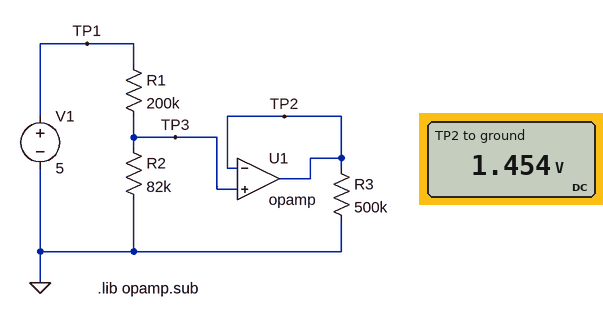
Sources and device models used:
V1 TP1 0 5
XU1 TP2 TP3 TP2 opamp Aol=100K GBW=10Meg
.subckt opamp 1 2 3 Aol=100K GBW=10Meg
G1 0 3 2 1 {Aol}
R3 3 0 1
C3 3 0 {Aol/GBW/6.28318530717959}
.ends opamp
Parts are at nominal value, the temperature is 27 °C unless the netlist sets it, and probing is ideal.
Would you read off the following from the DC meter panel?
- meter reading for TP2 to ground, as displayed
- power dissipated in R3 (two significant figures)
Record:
1.454 V
4.2 µW
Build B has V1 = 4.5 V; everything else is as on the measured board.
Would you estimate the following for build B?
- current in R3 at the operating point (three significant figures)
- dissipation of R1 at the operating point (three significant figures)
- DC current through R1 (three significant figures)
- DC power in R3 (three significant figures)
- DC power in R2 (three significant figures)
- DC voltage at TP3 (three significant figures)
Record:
2.62 µA
50.9 µW
16.0 µA
3.42 µW
20.9 µW
1.31 V
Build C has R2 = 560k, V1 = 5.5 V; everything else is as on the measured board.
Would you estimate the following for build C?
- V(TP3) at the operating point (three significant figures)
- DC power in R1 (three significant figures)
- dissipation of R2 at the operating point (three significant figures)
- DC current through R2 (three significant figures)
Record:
4.05 V
10.5 µW
29.3 µW
7.24 µA
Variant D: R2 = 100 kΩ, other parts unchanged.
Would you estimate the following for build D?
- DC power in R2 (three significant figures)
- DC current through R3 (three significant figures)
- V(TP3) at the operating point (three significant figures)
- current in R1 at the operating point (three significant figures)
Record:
27.8 µW
3.33 µA
1.67 V
16.7 µA
